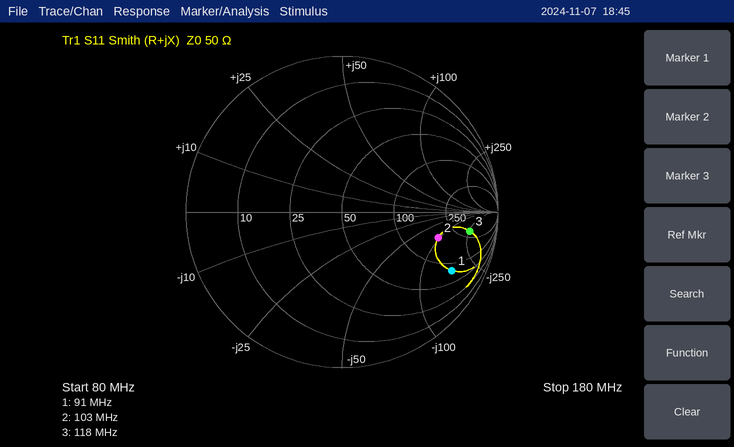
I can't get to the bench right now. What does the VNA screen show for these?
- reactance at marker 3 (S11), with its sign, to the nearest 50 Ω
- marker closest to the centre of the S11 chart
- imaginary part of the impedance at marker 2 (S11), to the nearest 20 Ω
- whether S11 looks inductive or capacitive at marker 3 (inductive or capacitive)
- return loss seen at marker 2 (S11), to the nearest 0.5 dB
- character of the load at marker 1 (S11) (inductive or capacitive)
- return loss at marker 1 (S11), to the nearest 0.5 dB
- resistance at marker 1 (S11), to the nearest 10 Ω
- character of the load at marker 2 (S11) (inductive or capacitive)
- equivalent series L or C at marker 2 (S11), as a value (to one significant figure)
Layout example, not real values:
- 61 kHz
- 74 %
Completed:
- -250 Ω
- marker 2
- -100 Ω
- capacitive
- 4.0 dB
- capacitive
- 2.0 dB
- 80 Ω
- capacitive
- 20 pF
